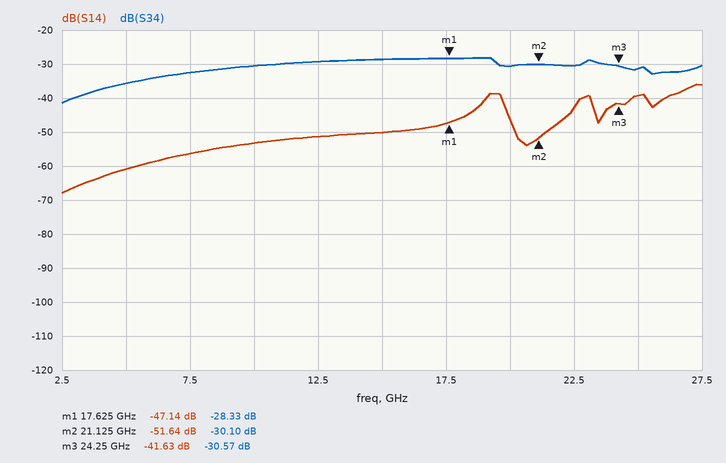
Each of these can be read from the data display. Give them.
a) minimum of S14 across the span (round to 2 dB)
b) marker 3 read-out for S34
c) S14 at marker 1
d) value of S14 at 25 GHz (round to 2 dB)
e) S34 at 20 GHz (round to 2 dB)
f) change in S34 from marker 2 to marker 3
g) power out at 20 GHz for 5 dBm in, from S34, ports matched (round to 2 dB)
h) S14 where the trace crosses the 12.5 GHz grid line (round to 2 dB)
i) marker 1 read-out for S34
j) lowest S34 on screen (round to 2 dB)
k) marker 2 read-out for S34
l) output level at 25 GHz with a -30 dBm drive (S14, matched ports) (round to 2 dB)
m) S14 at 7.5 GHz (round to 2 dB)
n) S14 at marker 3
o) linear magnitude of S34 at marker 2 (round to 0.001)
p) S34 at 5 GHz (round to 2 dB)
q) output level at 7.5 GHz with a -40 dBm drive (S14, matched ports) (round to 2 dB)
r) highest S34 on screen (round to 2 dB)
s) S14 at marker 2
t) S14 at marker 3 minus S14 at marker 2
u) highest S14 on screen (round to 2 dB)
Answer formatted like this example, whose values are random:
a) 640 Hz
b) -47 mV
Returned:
a) -68 dB
b) -30.57 dB
c) -47.14 dB
d) -40 dB
e) -30 dB
f) -0.47 dB
g) -26 dBm
h) -52 dB
i) -28.33 dB
j) -42 dB
k) -30.10 dB
l) -70 dBm
m) -56 dB
n) -41.63 dB
o) 0.031
p) -36 dB
q) -96 dBm
r) -28 dB
s) -51.64 dB
t) 10.01 dB
u) -36 dB
